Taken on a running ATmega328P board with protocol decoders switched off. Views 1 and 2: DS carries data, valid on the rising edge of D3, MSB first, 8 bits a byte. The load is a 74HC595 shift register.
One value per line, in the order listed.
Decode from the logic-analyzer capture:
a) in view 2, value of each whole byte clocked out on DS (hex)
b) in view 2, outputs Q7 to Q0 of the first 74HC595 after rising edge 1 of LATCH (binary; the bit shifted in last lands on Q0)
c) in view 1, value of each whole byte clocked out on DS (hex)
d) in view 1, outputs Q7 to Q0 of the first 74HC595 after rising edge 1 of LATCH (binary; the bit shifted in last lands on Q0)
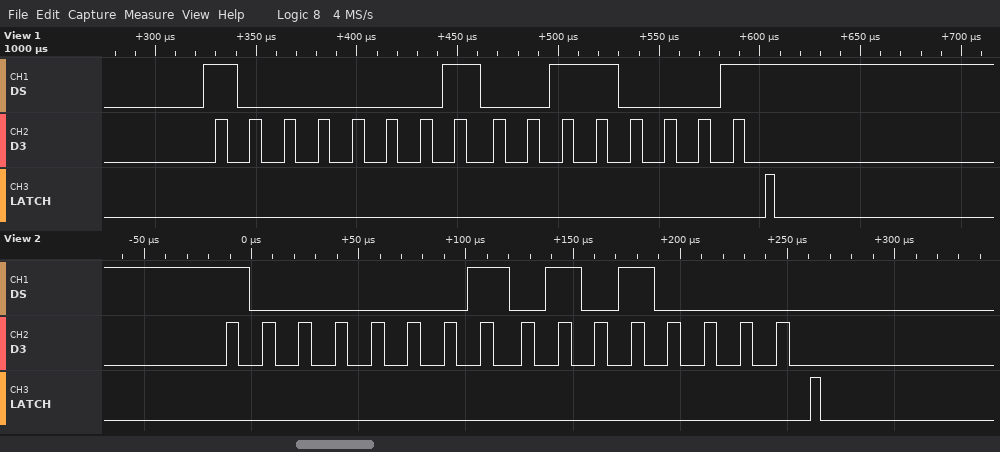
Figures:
81 50
01010000
81 31
00110001
